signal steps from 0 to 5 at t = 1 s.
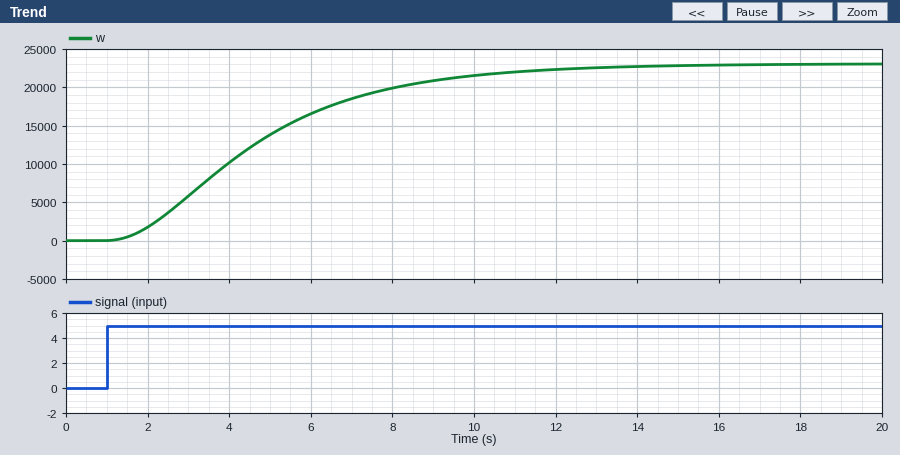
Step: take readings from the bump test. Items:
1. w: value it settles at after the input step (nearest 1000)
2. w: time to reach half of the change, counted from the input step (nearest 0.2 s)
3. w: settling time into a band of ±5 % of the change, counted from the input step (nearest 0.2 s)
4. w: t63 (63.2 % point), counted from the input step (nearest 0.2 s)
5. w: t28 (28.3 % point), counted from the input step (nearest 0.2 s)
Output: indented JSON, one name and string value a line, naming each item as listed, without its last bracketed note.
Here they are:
{
  "w: value it settles at after the input step": "23000",
  "w: time to reach half of the change, counted from the input step": "3.4 s",
  "w: settling time into a band of ±5 % of the change, counted from the input step": "9.8 s",
  "w: t63 (63.2 % point), counted from the input step": "4.2 s",
  "w: t28 (28.3 % point), counted from the input step": "2.2 s"
}
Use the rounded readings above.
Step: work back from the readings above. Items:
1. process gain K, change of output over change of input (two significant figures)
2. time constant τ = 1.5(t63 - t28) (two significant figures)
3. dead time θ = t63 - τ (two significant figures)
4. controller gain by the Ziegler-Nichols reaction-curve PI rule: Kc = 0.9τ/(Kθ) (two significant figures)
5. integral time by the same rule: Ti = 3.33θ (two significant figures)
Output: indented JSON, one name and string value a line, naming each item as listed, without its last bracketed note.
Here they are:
{
  "process gain K, change of output over change of input": "4600",
  "time constant τ = 1.5(t63 - t28)": "3.0 s",
  "dead time θ = t63 - τ": "1.2 s",
  "controller gain by the Ziegler-Nichols reaction-curve PI rule: Kc = 0.9τ/(Kθ)": "0.00049",
  "integral time by the same rule: Ti = 3.33θ": "4.0 s"
}
